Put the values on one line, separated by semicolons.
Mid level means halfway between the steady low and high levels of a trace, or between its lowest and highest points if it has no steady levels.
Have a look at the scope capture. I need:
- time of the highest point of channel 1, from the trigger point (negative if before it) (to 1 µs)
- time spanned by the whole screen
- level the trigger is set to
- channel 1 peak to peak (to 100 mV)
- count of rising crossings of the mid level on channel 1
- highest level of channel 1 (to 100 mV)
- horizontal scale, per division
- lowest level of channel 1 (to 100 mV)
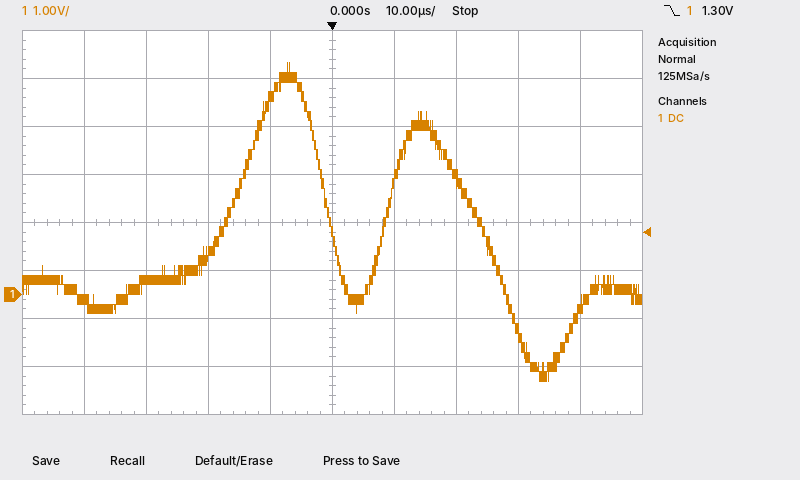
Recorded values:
-7 µs; 100 µs; 1.30 V; 6.6 V; 2; 4.8 V; 10 µs; -1.8 V
